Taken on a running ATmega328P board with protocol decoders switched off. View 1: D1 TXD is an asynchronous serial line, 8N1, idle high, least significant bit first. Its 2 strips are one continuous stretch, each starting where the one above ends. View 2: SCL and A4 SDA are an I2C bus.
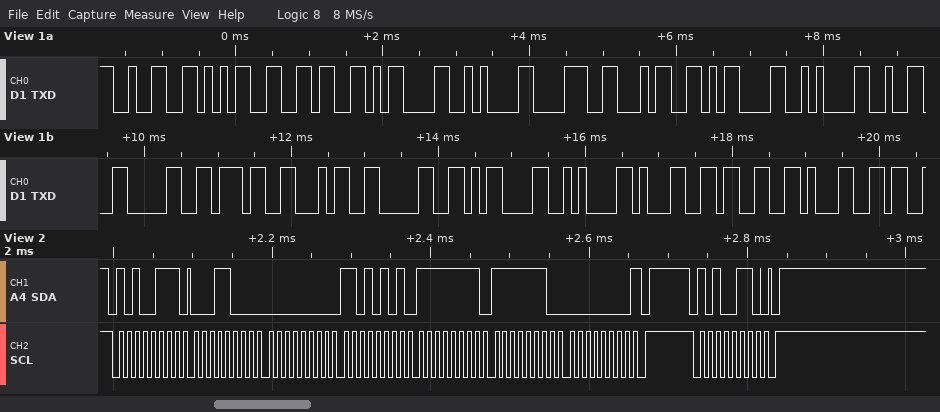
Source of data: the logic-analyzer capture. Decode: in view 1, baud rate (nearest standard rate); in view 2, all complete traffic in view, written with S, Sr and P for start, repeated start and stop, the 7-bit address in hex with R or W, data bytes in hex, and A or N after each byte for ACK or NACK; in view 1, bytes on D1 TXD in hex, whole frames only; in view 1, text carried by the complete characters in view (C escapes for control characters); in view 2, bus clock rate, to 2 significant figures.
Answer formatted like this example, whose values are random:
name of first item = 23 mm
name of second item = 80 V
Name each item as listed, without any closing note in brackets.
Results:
in view 1, baud rate = 9600 baud
in view 2, all complete traffic in view, written with S, Sr and P for start, repeated start and stop, the 7-bit address in hex with R or W, data bytes in hex, and A or N after each byte for ACK or NACK = S 53R A 18 A 00 A D5 A FF A FE A 00 N P S 53W A P
in view 1, bytes on D1 TXD in hex, whole frames only = 32 35 36 0D 0A 38 34 0D 0A 32 30 37 34 30 0D 0A 31 33 31
in view 1, text carried by the complete characters in view = "256\r\n84\r\n20740\r\n131"
in view 2, bus clock rate, to 2 significant figures = 100 kHz
